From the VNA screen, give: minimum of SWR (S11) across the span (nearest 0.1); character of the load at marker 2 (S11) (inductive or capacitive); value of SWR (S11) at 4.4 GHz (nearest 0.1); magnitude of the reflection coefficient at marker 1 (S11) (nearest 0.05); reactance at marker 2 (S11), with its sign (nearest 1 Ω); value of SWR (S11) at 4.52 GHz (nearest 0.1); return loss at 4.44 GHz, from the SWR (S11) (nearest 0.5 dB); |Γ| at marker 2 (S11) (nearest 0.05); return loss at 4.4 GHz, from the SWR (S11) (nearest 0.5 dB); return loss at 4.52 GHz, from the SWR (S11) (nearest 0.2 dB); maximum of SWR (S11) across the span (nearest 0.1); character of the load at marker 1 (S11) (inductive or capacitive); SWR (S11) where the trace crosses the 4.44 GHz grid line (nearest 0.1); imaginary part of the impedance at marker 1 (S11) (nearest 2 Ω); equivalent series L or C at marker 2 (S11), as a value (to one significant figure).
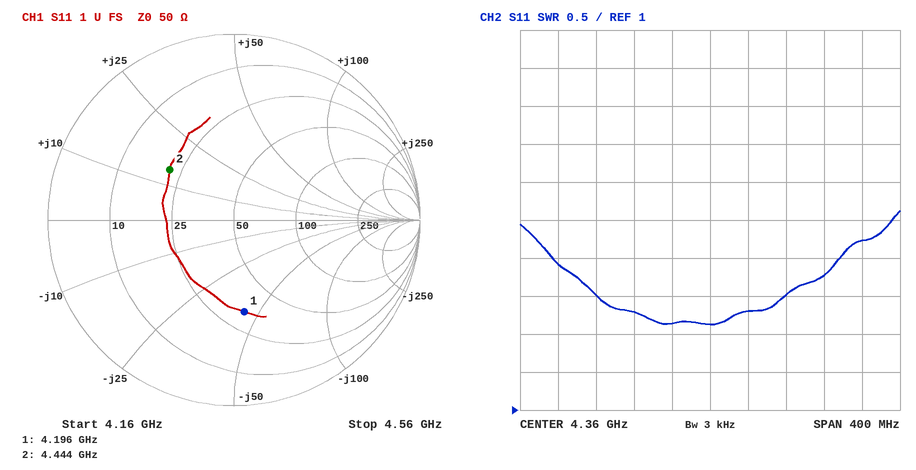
2.1
inductive
2.3
0.50
+14 Ω
3.2
7.5 dB
0.45
8.0 dB
5.6 dB
3.6
capacitive
2.5
-44 Ω
500 pH
